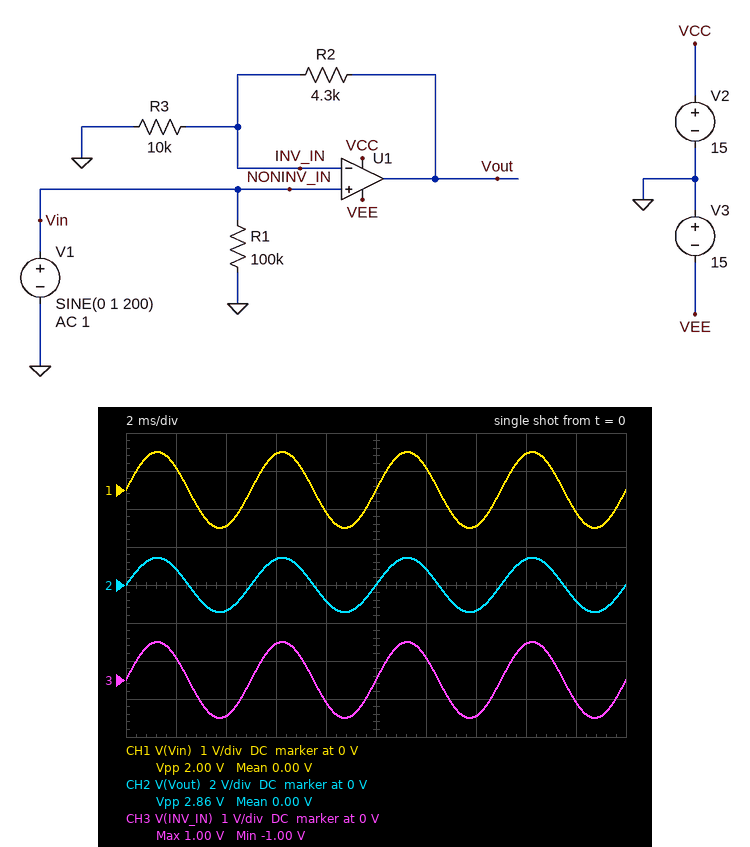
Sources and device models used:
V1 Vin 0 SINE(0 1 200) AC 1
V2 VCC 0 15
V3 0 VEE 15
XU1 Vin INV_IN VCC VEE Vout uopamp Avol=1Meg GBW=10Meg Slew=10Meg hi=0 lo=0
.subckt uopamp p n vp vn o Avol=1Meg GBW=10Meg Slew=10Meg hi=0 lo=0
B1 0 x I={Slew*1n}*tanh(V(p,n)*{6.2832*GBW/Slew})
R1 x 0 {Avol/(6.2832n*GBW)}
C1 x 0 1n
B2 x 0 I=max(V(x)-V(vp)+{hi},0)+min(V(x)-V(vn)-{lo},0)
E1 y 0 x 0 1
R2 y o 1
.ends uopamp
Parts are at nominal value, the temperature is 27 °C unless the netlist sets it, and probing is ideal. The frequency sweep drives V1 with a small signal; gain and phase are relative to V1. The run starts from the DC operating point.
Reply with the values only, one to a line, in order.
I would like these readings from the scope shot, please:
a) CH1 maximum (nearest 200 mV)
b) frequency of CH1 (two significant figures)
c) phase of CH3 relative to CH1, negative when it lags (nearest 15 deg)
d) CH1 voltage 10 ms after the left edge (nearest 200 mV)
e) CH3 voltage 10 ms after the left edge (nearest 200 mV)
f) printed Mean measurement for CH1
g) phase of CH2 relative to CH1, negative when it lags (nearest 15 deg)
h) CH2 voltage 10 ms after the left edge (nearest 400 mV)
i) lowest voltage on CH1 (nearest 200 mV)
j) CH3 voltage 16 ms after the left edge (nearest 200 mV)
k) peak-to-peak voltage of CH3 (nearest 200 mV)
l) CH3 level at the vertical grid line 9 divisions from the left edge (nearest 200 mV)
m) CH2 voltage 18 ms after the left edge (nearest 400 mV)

1.0 V
200 Hz
0 deg
0 V
0 V
0.00 V
0 deg
0 V
-1.0 V
1.0 V
2.0 V
-600 mV
-800 mV
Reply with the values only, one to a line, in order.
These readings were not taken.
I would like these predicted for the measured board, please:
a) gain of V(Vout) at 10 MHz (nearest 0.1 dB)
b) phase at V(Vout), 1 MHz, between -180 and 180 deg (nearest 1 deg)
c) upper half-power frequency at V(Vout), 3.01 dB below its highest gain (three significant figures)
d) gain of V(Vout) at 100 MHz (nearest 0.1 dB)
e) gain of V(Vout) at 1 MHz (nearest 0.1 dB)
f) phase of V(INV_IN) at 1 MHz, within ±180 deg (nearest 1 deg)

-1.7 dB
-8 deg
6.99 MHz
-20.0 dB
3.0 dB
-8 deg
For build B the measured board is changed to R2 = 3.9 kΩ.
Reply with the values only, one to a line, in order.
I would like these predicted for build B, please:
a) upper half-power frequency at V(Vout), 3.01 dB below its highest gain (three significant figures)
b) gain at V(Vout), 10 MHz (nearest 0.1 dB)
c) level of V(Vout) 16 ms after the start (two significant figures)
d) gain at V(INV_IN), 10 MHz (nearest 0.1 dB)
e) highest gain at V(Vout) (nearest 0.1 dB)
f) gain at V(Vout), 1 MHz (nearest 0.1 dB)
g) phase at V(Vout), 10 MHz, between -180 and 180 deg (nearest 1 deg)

7.19 MHz
-1.8 dB
1.3 V
-4.7 dB
2.9 dB
2.8 dB
-54 deg
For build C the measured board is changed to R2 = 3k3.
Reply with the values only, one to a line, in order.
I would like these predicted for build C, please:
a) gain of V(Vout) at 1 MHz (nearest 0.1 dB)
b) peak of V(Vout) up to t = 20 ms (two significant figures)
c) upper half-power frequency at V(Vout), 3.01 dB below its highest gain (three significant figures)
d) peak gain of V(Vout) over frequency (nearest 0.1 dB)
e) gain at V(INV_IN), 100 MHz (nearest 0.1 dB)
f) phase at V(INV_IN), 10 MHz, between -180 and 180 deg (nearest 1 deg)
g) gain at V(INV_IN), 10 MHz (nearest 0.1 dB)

2.4 dB
1.3 V
7.52 MHz
2.5 dB
-22.5 dB
-53 deg
-4.4 dB
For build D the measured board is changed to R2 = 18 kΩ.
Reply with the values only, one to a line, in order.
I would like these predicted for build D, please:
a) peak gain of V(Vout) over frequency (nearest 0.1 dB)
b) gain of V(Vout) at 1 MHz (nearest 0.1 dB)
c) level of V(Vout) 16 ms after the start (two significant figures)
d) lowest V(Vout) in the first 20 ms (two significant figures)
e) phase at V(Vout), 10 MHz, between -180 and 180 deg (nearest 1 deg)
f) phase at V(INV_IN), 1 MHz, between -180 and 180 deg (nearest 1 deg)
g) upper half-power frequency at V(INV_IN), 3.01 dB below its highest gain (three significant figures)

8.9 dB
8.6 dB
2.7 V
-2.8 V
-70 deg
-16 deg
3.57 MHz
